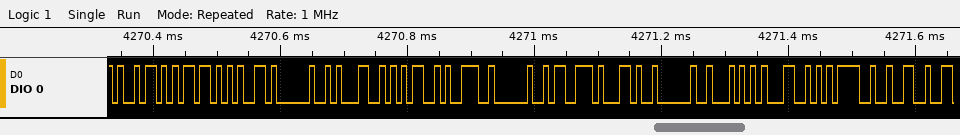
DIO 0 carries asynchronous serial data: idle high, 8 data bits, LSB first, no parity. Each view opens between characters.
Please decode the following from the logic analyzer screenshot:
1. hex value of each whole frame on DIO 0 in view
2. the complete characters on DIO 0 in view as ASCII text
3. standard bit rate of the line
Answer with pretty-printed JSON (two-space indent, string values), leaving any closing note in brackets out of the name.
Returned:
{
  "hex value of each whole frame on DIO 0 in view": "69, 6D, 65, 20, 31, 35, 39, 20, 73, 2C, 20, 54, 4C, 3D, 32",
  "the complete characters on DIO 0 in view as ASCII text": "\"ime 159 s, TL=2\"",
  "standard bit rate of the line": "115200 baud"
}
